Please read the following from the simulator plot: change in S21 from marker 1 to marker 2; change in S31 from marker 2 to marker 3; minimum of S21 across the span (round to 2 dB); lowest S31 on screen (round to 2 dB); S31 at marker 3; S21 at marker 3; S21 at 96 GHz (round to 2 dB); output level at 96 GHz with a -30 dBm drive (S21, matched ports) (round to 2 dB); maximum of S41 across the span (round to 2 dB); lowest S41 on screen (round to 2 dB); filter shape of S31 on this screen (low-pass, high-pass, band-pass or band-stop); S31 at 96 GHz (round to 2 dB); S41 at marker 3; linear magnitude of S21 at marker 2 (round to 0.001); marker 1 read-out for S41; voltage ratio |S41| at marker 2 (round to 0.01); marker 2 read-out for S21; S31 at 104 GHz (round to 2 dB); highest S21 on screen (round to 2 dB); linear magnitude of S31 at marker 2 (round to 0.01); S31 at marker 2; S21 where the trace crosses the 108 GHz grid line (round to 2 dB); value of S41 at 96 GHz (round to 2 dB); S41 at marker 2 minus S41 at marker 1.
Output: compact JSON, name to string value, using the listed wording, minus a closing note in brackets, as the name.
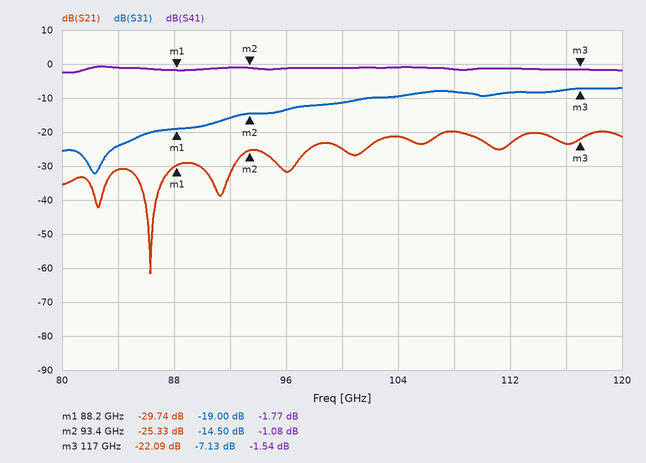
{"change in S21 from marker 1 to marker 2": "4.41 dB", "change in S31 from marker 2 to marker 3": "7.37 dB", "minimum of S21 across the span": "-62 dB", "lowest S31 on screen": "-32 dB", "S31 at marker 3": "-7.13 dB", "S21 at marker 3": "-22.09 dB", "S21 at 96 GHz": "-32 dB", "output level at 96 GHz with a -30 dBm drive (S21, matched ports)": "-62 dBm", "maximum of S41 across the span": "0 dB", "lowest S41 on screen": "-2 dB", "filter shape of S31 on this screen": "high-pass", "S31 at 96 GHz": "-14 dB", "S41 at marker 3": "-1.54 dB", "linear magnitude of S21 at marker 2": "0.054", "marker 1 read-out for S41": "-1.77 dB", "voltage ratio |S41| at marker 2": "0.88", "marker 2 read-out for S21": "-25.33 dB", "S31 at 104 GHz": "-10 dB", "highest S21 on screen": "-20 dB", "linear magnitude of S31 at marker 2": "0.19", "S31 at marker 2": "-14.50 dB", "S21 where the trace crosses the 108 GHz grid line": "-20 dB", "value of S41 at 96 GHz": "-2 dB", "S41 at marker 2 minus S41 at marker 1": "0.69 dB"}
